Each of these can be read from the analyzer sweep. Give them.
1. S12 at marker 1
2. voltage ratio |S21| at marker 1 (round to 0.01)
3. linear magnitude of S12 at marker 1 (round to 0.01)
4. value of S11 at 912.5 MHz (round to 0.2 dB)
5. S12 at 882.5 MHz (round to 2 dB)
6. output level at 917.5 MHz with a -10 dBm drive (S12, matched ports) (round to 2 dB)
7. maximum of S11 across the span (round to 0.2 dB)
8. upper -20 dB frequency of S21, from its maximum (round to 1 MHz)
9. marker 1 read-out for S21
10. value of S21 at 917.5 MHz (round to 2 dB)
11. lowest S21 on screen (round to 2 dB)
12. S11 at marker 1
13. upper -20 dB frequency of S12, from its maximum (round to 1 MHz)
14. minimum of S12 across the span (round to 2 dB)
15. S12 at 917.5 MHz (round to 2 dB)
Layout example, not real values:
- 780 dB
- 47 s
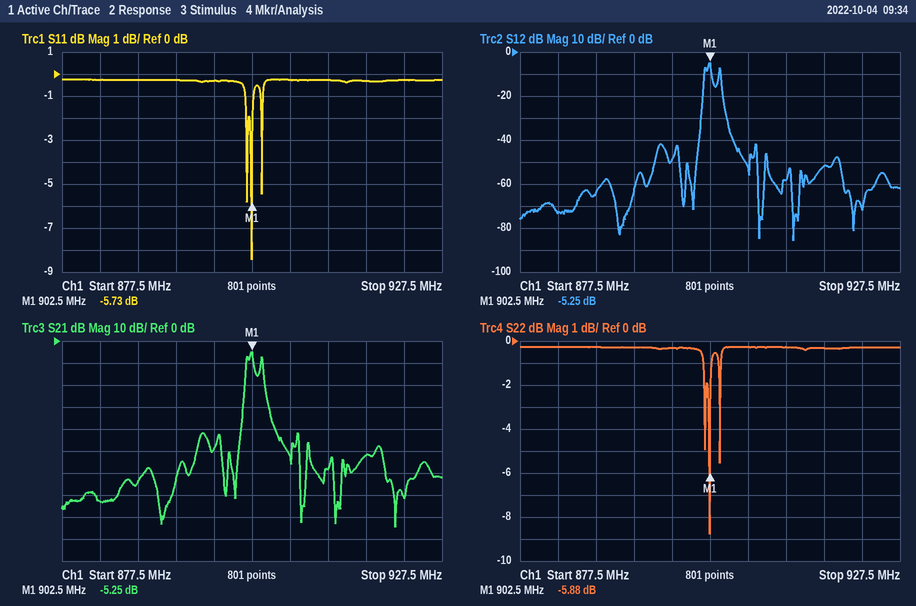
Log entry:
- -5.25 dB
- 0.55
- 0.55
- -0.2 dB
- -72 dB
- -62 dBm
- -0.2 dB
- 904 MHz
- -5.25 dB
- -52 dB
- -84 dB
- -5.73 dB
- 904 MHz
- -86 dB
- -52 dB
